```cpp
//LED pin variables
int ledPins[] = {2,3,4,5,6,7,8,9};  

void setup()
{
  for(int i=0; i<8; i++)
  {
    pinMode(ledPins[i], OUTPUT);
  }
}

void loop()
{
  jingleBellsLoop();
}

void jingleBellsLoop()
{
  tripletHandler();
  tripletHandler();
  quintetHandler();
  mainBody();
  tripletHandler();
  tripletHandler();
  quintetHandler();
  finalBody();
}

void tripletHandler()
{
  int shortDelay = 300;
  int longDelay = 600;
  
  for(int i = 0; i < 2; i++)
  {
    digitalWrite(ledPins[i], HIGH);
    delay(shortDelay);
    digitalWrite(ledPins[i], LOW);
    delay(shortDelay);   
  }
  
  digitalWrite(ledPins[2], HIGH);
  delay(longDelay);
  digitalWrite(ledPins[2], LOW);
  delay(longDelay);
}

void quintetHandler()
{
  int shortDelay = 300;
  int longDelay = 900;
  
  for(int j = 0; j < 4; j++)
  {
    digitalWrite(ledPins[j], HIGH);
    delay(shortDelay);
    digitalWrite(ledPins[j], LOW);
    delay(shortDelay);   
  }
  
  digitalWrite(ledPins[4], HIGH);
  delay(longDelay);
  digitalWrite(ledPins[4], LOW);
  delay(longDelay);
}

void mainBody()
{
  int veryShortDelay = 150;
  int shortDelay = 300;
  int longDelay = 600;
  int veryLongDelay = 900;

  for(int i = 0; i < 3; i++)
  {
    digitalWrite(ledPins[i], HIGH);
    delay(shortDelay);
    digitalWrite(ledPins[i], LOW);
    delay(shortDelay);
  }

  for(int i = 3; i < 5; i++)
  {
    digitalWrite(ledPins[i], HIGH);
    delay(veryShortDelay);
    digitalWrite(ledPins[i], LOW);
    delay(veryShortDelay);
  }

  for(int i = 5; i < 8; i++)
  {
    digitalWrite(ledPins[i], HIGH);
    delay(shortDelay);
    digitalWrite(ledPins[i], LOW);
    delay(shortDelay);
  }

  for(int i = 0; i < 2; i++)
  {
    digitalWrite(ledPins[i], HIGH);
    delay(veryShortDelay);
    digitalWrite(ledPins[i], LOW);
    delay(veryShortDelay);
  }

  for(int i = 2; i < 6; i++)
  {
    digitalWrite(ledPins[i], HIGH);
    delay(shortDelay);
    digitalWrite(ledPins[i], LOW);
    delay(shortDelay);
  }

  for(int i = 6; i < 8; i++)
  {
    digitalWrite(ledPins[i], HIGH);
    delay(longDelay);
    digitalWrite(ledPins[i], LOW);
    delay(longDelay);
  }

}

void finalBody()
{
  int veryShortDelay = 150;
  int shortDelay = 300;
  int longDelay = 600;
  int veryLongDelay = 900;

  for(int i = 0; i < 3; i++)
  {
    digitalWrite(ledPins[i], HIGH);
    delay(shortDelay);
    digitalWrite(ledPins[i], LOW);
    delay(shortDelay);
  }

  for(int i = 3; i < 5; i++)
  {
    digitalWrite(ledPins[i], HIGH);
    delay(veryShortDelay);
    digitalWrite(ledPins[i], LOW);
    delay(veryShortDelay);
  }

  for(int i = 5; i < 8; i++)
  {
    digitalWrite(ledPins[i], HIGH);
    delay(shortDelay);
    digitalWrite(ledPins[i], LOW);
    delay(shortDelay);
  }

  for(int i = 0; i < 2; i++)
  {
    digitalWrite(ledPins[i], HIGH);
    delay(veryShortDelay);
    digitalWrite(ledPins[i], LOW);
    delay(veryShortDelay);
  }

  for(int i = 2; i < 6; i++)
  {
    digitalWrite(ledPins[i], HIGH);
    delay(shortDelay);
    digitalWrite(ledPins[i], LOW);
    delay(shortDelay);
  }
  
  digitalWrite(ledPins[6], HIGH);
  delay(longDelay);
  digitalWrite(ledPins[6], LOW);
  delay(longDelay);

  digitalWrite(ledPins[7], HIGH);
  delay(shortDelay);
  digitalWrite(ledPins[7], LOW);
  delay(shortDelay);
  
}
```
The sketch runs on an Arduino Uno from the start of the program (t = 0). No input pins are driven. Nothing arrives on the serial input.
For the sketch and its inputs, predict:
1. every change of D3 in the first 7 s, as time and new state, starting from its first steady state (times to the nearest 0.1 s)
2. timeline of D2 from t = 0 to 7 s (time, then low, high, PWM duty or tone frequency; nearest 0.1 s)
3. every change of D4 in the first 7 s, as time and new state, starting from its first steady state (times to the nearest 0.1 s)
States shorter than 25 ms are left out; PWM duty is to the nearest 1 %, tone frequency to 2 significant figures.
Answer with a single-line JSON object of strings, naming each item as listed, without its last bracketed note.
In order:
{"every change of D3 in the first 7 s, as time and new state, starting from its first steady state": "0 s low; 0.6 s high; 0.9 s low; 3 s high; 3.3 s low; 5.4 s high; 5.7 s low", "timeline of D2 from t = 0 to 7 s": "0 s high; 0.3 s low; 2.4 s high; 2.7 s low; 4.8 s high; 5.1 s low", "every change of D4 in the first 7 s, as time and new state, starting from its first steady state": "0 s low; 1.2 s high; 1.8 s low; 3.6 s high; 4.2 s low; 6 s high; 6.3 s low"}
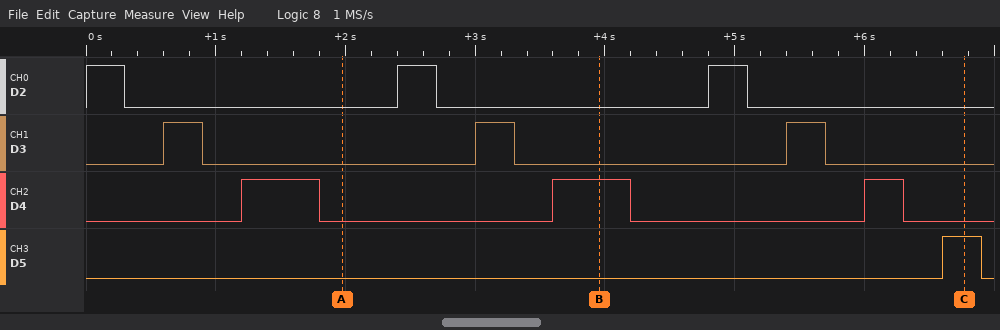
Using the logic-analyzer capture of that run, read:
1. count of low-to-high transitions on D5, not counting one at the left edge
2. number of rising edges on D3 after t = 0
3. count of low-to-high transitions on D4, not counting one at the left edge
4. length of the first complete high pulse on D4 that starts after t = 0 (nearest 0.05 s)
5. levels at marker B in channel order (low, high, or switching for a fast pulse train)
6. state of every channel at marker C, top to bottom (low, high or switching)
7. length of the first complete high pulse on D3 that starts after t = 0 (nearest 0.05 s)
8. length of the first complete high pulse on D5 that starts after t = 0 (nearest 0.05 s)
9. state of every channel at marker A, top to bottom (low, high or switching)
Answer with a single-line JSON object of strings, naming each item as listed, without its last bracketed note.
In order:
{"count of low-to-high transitions on D5, not counting one at the left edge": "1", "number of rising edges on D3 after t = 0": "3", "count of low-to-high transitions on D4, not counting one at the left edge": "3", "length of the first complete high pulse on D4 that starts after t = 0": "0.60 s", "levels at marker B in channel order": "D2 low, D3 low, D4 high, D5 low", "state of every channel at marker C, top to bottom": "D2 low, D3 low, D4 low, D5 high", "length of the first complete high pulse on D3 that starts after t = 0": "0.30 s", "length of the first complete high pulse on D5 that starts after t = 0": "0.30 s", "state of every channel at marker A, top to bottom": "D2 low, D3 low, D4 low, D5 low"}
